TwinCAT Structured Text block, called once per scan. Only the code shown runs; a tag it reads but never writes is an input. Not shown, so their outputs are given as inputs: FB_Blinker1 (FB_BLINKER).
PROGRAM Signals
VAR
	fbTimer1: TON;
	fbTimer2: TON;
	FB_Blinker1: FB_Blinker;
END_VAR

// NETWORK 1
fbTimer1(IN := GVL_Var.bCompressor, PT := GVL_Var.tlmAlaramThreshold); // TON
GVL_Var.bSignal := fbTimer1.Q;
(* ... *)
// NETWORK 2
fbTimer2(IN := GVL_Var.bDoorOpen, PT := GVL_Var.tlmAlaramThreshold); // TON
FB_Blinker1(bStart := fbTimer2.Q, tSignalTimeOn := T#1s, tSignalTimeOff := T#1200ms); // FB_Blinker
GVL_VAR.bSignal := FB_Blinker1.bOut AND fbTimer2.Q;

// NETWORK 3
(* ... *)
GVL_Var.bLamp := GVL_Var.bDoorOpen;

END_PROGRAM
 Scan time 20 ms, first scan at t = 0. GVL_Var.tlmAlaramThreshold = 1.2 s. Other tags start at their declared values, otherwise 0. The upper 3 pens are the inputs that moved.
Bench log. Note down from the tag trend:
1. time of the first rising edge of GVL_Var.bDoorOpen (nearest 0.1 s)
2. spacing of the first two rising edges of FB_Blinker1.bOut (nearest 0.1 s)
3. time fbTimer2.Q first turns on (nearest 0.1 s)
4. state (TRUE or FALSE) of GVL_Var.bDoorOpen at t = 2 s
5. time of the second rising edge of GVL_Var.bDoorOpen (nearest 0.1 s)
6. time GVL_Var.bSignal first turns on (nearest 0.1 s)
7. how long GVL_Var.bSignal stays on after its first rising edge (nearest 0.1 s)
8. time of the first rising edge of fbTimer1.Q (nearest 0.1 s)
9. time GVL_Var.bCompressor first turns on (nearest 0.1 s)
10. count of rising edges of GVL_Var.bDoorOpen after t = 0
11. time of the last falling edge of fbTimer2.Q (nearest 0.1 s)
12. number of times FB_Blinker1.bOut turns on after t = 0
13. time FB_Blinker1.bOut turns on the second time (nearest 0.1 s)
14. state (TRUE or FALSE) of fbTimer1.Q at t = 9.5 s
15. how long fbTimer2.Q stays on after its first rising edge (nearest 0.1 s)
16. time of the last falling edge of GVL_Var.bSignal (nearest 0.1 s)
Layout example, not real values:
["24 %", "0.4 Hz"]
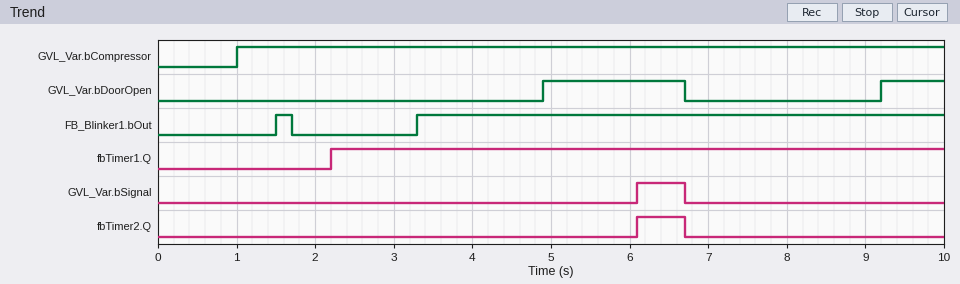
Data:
["4.9 s", "1.8 s", "6.1 s", "FALSE", "9.2 s", "6.1 s", "0.6 s", "2.2 s", "1.0 s", "2", "6.7 s", "2", "3.3 s", "TRUE", "0.6 s", "6.7 s"]
